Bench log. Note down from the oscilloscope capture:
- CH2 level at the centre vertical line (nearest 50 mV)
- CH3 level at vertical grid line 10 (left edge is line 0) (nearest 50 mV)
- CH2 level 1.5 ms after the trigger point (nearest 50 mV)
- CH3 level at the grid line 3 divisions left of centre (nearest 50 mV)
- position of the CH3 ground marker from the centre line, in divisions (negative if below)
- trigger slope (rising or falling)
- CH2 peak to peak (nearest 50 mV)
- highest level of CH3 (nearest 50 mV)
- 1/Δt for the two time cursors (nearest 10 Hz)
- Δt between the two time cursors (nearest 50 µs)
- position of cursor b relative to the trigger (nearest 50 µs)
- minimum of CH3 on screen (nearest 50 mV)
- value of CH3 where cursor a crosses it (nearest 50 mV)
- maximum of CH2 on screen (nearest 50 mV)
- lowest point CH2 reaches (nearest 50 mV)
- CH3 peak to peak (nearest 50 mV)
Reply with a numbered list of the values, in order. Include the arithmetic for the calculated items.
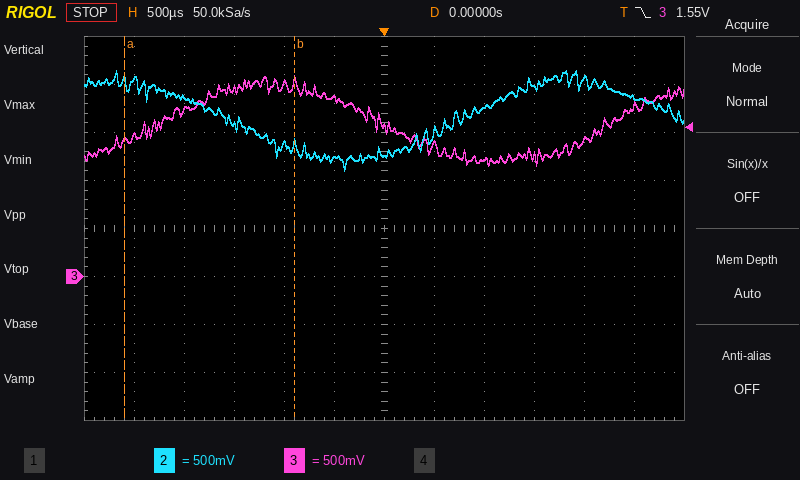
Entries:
1. 1.25 V
2. 1.40 V
3. 1.95 V
4. 1.95 V
5. -1.0 div
6. falling
7. 2.15 V − (1.10 V) = 1.05 V
8. 2.10 V
9. 1 / 1.70 ms ≈ 590 Hz
10. 1.70 ms
11. -900 µs
12. 1.15 V
13. 1.40 V
14. 2.15 V
15. 1.10 V
16. 2.10 V − (1.15 V) = 950 mV
